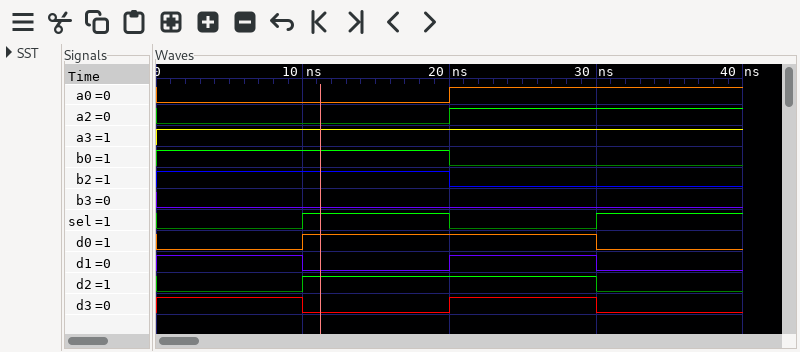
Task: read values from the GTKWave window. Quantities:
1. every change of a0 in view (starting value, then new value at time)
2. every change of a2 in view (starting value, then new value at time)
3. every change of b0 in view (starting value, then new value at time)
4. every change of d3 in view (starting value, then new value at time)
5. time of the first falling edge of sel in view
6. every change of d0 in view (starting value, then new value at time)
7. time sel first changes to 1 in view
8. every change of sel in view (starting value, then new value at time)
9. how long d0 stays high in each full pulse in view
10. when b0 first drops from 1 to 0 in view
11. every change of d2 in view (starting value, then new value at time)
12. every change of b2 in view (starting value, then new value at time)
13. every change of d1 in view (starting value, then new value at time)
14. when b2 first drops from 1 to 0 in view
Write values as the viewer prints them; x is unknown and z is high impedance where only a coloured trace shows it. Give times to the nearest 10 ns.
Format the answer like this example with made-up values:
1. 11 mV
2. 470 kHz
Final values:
1. 0, 1 at 20 ns
2. 0, 1 at 20 ns
3. 1, 0 at 20 ns
4. 1, 0 at 10 ns, 1 at 20 ns, 0 at 30 ns
5. 20 ns
6. 0, 1 at 10 ns, 0 at 30 ns
7. 10 ns
8. 0, 1 at 10 ns, 0 at 20 ns, 1 at 30 ns
9. 20 ns
10. 20 ns
11. 0, 1 at 10 ns, 0 at 30 ns
12. 1, 0 at 20 ns
13. 1, 0 at 10 ns, 1 at 20 ns, 0 at 30 ns
14. 20 ns
